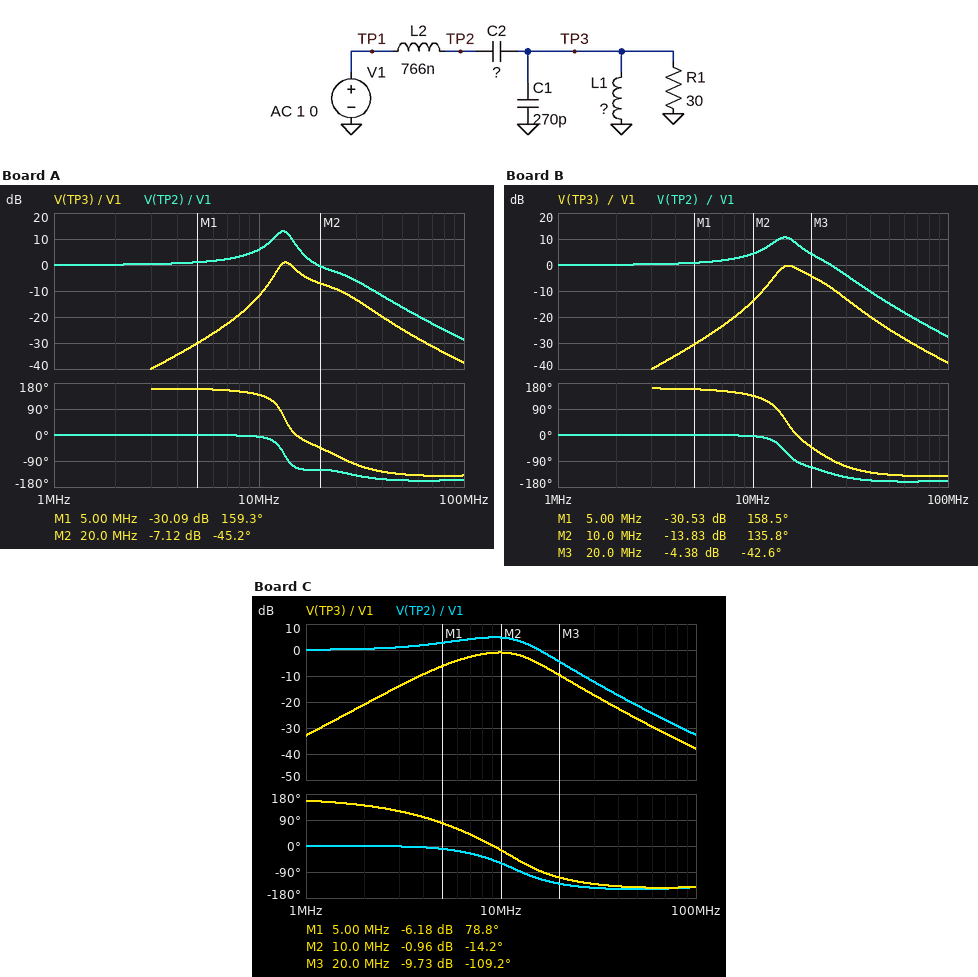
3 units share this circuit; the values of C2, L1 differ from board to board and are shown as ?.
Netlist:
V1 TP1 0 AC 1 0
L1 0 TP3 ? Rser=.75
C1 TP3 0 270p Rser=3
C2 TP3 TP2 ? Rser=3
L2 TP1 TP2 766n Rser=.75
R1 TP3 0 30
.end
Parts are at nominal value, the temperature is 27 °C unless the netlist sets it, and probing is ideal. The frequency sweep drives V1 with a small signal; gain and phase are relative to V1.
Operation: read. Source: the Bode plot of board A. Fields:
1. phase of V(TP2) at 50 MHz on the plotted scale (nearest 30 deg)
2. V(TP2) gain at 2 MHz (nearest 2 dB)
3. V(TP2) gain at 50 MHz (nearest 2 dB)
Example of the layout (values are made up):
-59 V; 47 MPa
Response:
-150 deg; 0 dB; -16 dB
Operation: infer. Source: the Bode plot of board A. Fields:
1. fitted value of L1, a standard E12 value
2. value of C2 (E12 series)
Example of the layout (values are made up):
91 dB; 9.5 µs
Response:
180 nH; 150 pF
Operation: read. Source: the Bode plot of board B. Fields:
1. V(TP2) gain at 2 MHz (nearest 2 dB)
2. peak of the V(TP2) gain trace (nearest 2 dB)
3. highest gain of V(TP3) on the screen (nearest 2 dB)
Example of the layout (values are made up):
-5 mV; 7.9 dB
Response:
0 dB; 10 dB; 0 dB
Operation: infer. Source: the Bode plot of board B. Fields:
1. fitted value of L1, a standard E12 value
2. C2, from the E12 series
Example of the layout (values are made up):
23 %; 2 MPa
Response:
220 nH; 120 pF
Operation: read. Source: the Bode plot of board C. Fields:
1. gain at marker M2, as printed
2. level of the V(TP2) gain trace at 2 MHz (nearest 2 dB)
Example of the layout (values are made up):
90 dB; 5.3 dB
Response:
-0.96 dB; 0 dB
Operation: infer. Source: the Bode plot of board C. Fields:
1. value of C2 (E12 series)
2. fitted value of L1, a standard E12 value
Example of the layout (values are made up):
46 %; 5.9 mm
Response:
390 pF; 1.5 µH
